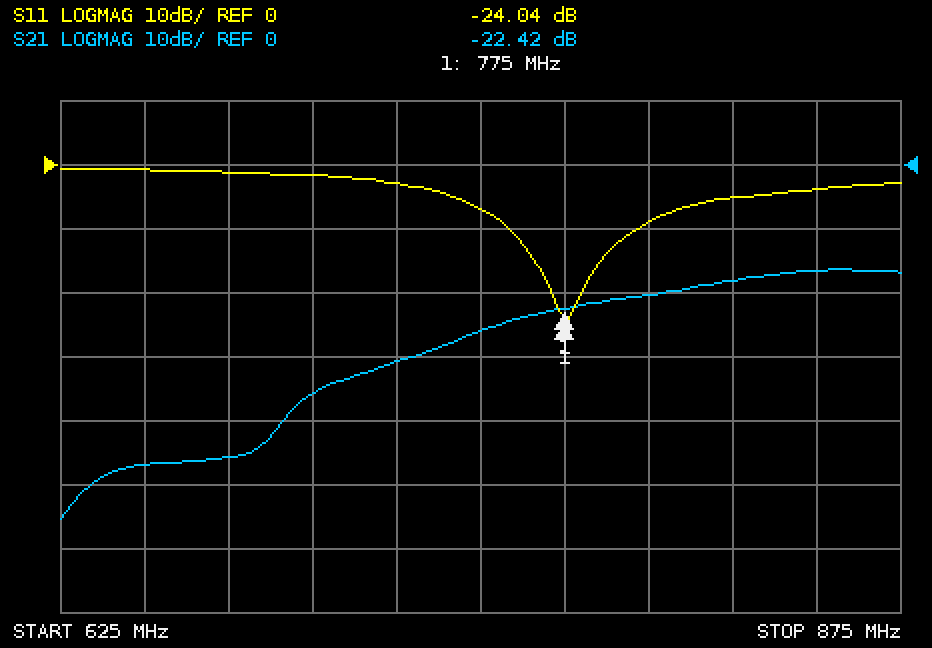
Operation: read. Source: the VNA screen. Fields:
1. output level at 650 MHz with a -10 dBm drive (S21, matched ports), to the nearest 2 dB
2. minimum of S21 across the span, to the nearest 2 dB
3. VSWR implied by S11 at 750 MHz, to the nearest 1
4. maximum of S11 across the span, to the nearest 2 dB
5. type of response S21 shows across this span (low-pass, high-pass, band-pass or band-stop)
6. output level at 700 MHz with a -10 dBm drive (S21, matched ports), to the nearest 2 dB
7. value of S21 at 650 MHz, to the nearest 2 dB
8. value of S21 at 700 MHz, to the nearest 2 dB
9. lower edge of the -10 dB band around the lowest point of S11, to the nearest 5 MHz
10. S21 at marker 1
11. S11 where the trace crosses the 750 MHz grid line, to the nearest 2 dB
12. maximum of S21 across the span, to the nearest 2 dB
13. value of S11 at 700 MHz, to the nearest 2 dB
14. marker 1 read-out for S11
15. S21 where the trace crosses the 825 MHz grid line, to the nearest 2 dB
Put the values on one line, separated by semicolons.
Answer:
-56 dBm; -56 dB; 3; 0 dB; high-pass; -46 dBm; -46 dB; -36 dB; 760 MHz; -22.42 dB; -6 dB; -16 dB; -2 dB; -24.04 dB; -18 dB
